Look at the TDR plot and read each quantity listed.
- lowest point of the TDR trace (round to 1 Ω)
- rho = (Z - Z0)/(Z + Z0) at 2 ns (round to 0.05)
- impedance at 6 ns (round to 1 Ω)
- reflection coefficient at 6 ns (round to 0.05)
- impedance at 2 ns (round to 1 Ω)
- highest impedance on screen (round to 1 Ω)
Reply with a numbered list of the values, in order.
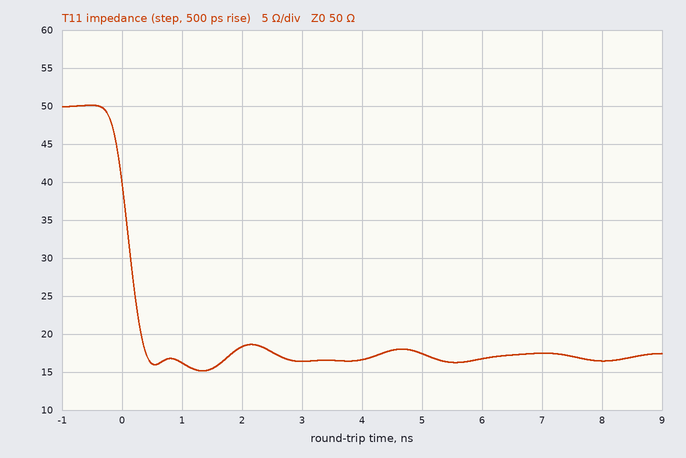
1. 15 Ω
2. -0.45
3. 17 Ω
4. -0.50
5. 18 Ω
6. 50 Ω
